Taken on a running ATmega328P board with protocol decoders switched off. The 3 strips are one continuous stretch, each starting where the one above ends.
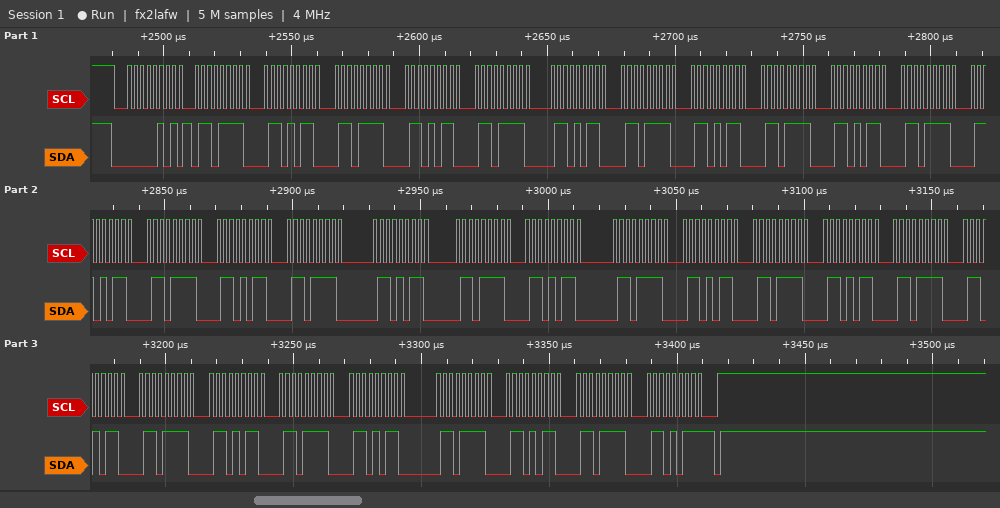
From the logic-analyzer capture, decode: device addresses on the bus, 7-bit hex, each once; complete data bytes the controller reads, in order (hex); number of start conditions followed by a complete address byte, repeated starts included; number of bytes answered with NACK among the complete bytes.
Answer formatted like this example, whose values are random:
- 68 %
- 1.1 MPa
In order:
- 0x02
- 6F 6B 6F 6B 6F 6B 6F 6B 6F 6B 6F 6B 6F 6B 6F 6B 6F 6B 6F 6B 6F 6B 6F 6B 6F 6B 6F 6B 6F 6B 6F 6B
- 1
- 1
